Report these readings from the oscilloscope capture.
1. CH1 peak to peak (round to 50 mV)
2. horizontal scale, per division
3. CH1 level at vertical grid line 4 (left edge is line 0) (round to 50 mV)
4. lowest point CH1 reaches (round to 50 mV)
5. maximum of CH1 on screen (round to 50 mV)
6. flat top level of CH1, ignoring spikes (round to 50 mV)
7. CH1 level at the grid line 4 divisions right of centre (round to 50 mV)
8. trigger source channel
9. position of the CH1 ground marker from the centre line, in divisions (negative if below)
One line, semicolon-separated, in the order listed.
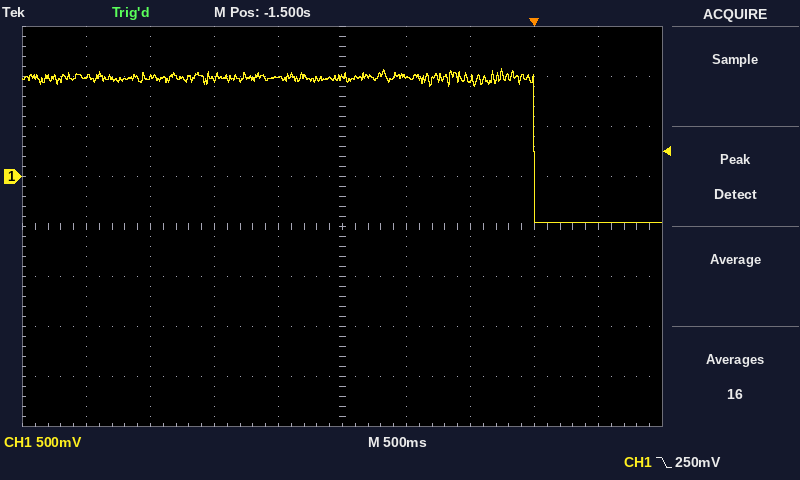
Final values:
1.55 V; 500 ms; 1.00 V; -450 mV; 1.10 V; 1.00 V; -450 mV; CH1; +1.0 div
